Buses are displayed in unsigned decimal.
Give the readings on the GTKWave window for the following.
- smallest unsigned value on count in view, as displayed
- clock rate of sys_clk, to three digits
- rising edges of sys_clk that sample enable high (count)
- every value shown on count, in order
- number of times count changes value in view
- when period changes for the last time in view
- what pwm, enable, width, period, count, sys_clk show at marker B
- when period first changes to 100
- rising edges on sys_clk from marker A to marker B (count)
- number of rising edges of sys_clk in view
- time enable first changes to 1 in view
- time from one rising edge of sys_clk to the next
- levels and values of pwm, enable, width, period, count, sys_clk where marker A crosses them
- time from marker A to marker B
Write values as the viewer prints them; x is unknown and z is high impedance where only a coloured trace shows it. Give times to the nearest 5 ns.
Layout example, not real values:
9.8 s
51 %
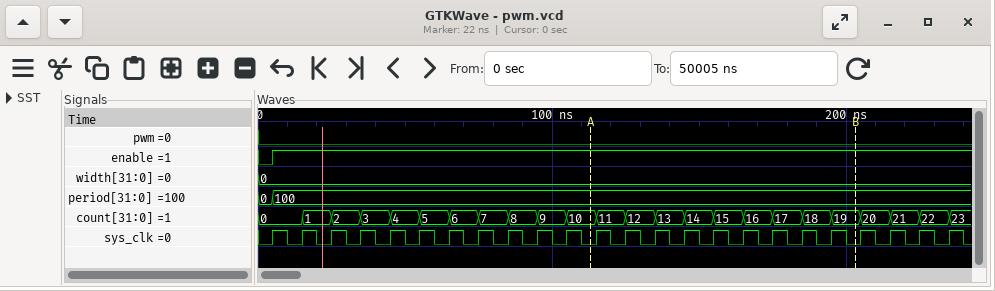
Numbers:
0
100 MHz
23
0, 1, 2, 3, 4, 5, 6, 7, 8, 9, 10, 11, 12, 13, 14, 15, 16, 17, 18, 19, 20, 21, 22, 23
23
5 ns
pwm=0, enable=1, width=0, period=100, count=19, sys_clk=0
5 ns
9
24
5 ns
10 ns
pwm=0, enable=1, width=0, period=100, count=10, sys_clk=0
90 ns
